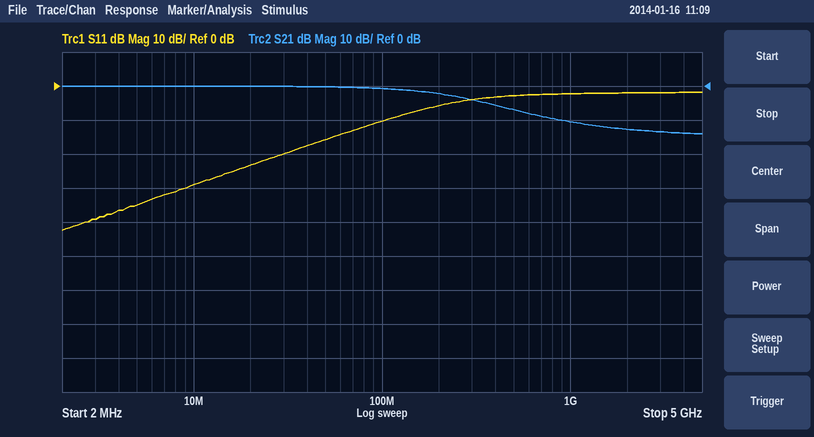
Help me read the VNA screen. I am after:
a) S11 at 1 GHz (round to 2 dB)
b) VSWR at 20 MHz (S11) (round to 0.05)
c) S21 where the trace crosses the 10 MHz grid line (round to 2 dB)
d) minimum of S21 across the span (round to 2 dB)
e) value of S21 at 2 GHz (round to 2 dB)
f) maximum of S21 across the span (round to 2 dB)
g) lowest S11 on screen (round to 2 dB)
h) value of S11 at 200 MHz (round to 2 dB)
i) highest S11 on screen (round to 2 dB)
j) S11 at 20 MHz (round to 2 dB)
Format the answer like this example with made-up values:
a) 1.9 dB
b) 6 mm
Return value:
a) -2 dB
b) 1.15
c) 0 dB
d) -14 dB
e) -12 dB
f) 0 dB
g) -42 dB
h) -6 dB
i) -2 dB
j) -24 dB
